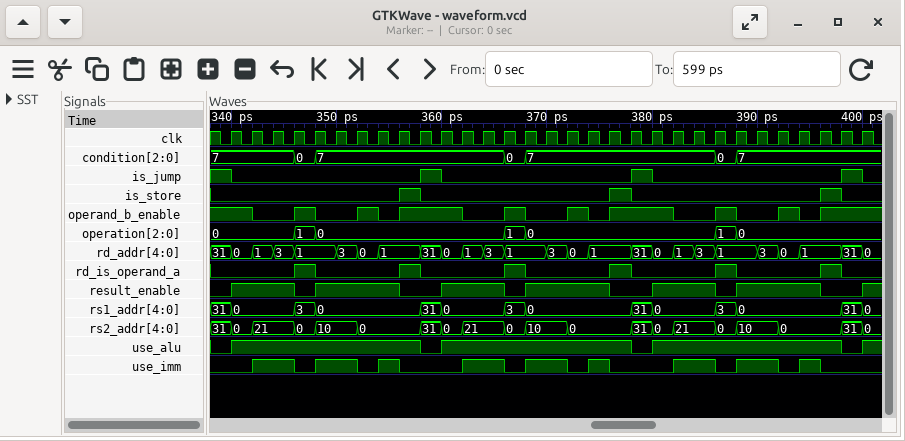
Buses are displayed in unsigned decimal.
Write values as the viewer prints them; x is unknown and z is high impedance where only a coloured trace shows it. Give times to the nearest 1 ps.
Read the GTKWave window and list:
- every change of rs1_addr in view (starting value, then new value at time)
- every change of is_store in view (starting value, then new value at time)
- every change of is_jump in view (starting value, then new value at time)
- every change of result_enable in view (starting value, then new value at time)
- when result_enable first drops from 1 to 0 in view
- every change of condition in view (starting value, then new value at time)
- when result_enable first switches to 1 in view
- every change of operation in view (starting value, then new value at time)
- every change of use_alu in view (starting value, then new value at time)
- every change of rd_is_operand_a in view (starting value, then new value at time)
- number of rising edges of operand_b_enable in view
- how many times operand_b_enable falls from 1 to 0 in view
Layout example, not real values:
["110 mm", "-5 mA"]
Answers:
["31, 0 at 340 ps, 3 at 346 ps, 0 at 348 ps, 31 at 358 ps, 0 at 360 ps, 3 at 366 ps, 0 at 368 ps, 31 at 378 ps, 0 at 380 ps, 3 at 386 ps, 0 at 388 ps, 31 at 398 ps, 0 at 400 ps", "0, 1 at 356 ps, 0 at 358 ps, 1 at 376 ps, 0 at 378 ps, 1 at 396 ps, 0 at 398 ps", "1, 0 at 340 ps, 1 at 358 ps, 0 at 360 ps, 1 at 378 ps, 0 at 380 ps, 1 at 398 ps, 0 at 400 ps", "0, 1 at 340 ps, 0 at 346 ps, 1 at 348 ps, 0 at 356 ps, 1 at 360 ps, 0 at 366 ps, 1 at 368 ps, 0 at 376 ps, 1 at 380 ps, 0 at 386 ps, 1 at 388 ps, 0 at 396 ps, 1 at 400 ps", "346 ps", "7, 0 at 346 ps, 7 at 348 ps, 0 at 366 ps, 7 at 368 ps, 0 at 386 ps, 7 at 388 ps", "340 ps", "0, 1 at 346 ps, 0 at 348 ps, 1 at 366 ps, 0 at 368 ps, 1 at 386 ps, 0 at 388 ps", "0, 1 at 340 ps, 0 at 358 ps, 1 at 360 ps, 0 at 378 ps, 1 at 380 ps, 0 at 398 ps, 1 at 400 ps", "0, 1 at 346 ps, 0 at 348 ps, 1 at 356 ps, 0 at 358 ps, 1 at 366 ps, 0 at 368 ps, 1 at 376 ps, 0 at 378 ps, 1 at 386 ps, 0 at 388 ps, 1 at 396 ps, 0 at 398 ps", "9", "9"]
